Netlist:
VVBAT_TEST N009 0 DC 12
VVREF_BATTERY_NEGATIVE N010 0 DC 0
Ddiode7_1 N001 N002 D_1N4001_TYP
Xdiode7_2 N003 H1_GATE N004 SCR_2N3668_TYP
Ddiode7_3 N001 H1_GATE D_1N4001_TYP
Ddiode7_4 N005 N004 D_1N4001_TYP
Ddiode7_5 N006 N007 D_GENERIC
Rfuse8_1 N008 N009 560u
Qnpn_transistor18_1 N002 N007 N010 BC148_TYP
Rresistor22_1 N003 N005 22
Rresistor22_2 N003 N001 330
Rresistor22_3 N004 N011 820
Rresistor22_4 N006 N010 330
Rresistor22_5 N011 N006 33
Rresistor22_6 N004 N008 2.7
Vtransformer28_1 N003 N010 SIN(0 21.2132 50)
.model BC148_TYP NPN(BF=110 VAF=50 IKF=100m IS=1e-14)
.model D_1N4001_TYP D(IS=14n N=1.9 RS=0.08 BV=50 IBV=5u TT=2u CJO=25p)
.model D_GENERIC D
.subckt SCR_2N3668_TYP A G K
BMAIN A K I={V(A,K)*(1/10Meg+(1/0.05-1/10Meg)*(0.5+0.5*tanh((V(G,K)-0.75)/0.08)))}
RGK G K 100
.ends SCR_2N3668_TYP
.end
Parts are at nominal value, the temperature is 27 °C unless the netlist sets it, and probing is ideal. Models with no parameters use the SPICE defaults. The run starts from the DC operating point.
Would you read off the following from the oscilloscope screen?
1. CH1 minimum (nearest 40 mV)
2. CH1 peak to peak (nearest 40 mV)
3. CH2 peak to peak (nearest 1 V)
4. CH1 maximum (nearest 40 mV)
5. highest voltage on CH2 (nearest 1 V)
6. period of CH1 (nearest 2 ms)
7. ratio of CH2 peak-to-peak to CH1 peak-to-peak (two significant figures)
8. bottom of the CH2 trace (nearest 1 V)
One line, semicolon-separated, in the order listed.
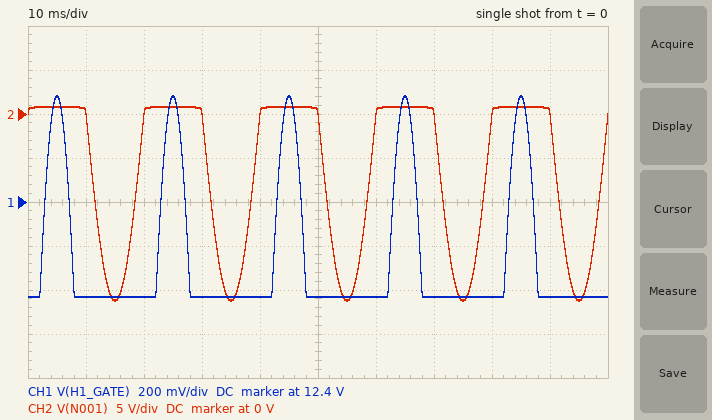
11.96 V; 920 mV; 22 V; 12.88 V; 1 V; 20 ms; 24; -21 V
